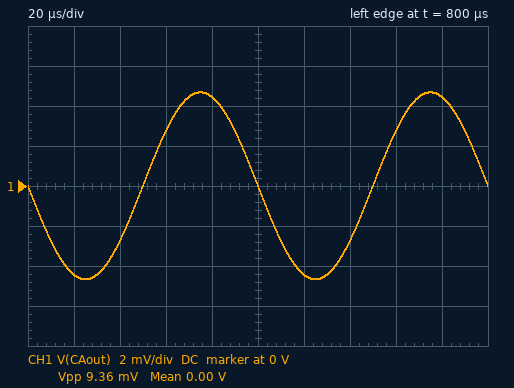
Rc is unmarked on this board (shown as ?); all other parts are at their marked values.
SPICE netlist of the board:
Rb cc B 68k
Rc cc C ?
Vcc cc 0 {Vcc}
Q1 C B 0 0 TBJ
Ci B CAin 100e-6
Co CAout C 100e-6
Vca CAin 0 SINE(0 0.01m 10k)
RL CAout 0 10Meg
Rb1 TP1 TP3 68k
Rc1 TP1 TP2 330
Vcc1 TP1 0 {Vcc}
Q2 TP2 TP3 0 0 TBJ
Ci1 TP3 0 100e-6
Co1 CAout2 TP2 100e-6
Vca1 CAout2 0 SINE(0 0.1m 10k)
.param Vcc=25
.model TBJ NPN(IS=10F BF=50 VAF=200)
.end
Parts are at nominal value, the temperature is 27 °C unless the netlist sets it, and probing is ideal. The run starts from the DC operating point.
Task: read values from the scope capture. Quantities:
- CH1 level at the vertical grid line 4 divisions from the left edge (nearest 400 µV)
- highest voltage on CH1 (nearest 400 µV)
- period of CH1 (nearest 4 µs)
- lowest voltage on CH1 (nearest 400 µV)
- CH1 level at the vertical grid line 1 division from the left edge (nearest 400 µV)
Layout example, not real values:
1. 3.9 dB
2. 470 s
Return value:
1. 4.4 mV
2. 4.8 mV
3. 100 µs
4. -4.8 mV
5. -4.4 mV
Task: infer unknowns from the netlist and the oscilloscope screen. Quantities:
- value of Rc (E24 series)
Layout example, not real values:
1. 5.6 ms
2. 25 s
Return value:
1. 680 Ω
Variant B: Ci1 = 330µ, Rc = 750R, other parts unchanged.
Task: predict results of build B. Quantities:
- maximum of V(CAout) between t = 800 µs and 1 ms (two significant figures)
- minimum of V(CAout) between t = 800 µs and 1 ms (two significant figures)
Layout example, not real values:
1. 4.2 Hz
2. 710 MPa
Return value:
1. 5.1 mV
2. -5.1 mV
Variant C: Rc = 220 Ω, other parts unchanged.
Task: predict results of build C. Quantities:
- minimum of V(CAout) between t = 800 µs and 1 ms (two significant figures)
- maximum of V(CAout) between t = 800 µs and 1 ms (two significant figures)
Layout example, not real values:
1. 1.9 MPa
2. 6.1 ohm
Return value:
1. -1.6 mV
2. 1.6 mV
